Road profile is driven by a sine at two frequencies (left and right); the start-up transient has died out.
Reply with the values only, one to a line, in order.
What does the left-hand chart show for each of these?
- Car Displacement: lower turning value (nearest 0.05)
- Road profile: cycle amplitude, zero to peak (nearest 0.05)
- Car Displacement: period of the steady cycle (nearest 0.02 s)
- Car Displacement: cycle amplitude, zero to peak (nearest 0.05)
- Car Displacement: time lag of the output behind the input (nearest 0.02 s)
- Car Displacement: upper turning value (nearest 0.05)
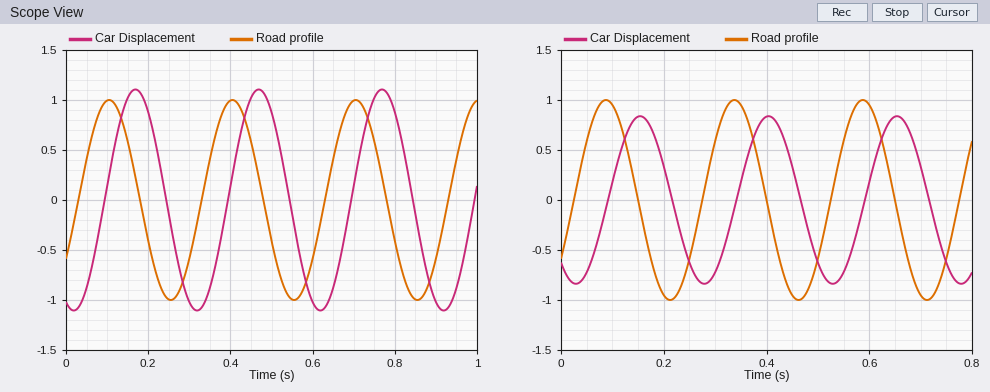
-1.10
1.00
0.30 s
1.10
0.06 s
1.10
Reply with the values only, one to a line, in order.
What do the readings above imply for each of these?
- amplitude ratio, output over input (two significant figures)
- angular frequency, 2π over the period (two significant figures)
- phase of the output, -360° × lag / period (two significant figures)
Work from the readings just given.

1.1
21 rad/s
-72°
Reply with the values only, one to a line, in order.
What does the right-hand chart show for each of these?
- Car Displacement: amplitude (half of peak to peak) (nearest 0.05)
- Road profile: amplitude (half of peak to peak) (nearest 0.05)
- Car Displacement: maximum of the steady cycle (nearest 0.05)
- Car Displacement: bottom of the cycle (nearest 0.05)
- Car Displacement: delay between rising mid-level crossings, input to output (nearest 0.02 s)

0.85
1.00
0.85
-0.85
0.06 s
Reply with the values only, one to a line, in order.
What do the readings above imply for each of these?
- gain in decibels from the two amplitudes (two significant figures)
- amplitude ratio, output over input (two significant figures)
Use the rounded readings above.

-1.4 dB
0.85
